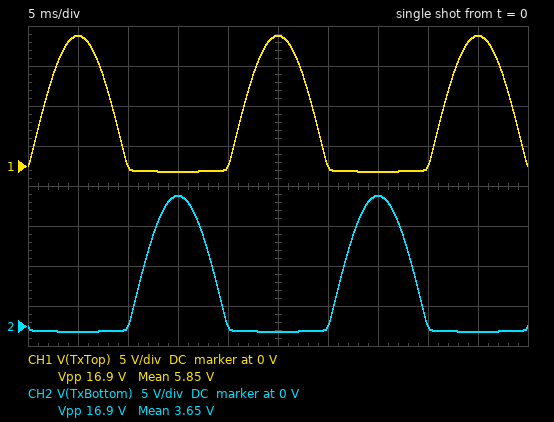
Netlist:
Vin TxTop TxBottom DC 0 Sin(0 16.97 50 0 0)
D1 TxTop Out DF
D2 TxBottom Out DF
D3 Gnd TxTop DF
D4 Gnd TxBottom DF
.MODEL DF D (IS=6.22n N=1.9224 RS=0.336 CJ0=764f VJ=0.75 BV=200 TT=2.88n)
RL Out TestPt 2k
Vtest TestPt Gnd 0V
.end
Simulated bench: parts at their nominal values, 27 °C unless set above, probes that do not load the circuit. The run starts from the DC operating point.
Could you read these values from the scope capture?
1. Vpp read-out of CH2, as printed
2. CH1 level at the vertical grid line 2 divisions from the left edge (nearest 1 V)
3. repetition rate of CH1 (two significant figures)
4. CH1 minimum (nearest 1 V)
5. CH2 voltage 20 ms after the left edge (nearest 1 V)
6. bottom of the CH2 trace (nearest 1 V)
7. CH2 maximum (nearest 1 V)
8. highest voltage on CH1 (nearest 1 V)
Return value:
16.9 V
0 V
50 Hz
-1 V
0 V
-1 V
16 V
16 V
